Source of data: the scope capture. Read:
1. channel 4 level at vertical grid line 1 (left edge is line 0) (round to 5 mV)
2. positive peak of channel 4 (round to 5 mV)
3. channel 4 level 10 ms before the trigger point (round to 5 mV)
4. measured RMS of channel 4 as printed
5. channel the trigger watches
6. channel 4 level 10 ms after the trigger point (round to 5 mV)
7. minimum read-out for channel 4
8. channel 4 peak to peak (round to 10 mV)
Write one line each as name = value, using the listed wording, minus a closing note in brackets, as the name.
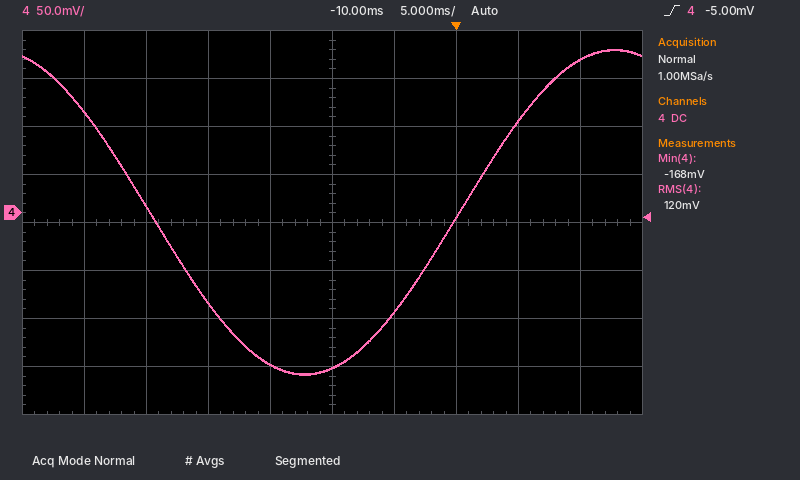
channel 4 level at vertical grid line 1 (left edge is line 0) = 105 mV
positive peak of channel 4 = 170 mV
channel 4 level 10 ms before the trigger point = -160 mV
measured RMS of channel 4 as printed = 120 mV
channel the trigger watches = channel 4
channel 4 level 10 ms after the trigger point = 160 mV
minimum read-out for channel 4 = -168 mV
channel 4 peak to peak = 340 mV
